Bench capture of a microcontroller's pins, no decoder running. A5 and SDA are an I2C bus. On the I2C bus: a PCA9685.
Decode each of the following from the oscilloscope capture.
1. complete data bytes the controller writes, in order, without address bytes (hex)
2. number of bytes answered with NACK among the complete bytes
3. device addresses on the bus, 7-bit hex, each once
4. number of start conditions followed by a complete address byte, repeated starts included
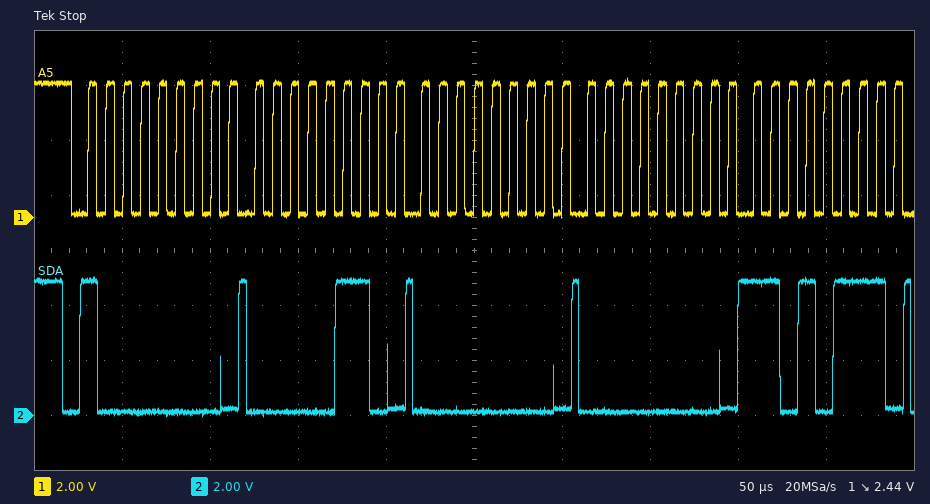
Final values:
06 00 00 D7
0
0x40
1
